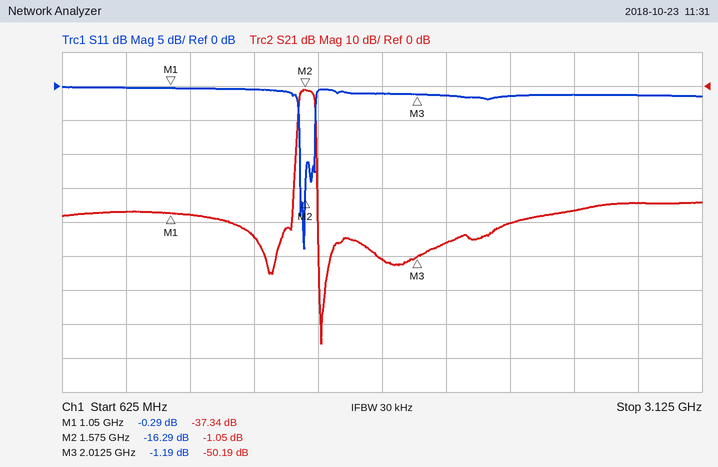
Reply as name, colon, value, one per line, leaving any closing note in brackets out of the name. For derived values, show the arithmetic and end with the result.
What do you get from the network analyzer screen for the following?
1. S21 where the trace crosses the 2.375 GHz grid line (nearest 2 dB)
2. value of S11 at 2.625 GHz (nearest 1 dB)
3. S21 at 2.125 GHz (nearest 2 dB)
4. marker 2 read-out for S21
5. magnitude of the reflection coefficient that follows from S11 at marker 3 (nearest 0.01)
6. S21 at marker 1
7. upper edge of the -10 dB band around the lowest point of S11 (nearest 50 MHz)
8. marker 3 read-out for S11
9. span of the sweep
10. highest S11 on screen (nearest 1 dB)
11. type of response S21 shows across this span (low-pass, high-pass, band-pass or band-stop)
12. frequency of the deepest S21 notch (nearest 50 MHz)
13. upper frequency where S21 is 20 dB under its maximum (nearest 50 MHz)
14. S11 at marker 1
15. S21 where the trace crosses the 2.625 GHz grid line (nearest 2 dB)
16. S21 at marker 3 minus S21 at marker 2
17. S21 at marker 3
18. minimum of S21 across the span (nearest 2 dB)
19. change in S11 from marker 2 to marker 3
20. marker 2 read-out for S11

S21 where the trace crosses the 2.375 GHz grid line: -40 dB
value of S11 at 2.625 GHz: -1 dB
S21 at 2.125 GHz: -46 dB
marker 2 read-out for S21: -1.05 dB
magnitude of the reflection coefficient that follows from S11 at marker 3: 10^(-1.19/20) ≈ 0.87
S21 at marker 1: -37.34 dB
upper edge of the -10 dB band around the lowest point of S11: 1.60 GHz
marker 3 read-out for S11: -1.19 dB
span of the sweep: 2.5 GHz
highest S11 on screen: 0 dB
type of response S21 shows across this span: band-pass
frequency of the deepest S21 notch: 1.65 GHz
upper frequency where S21 is 20 dB under its maximum: 1.60 GHz
S11 at marker 1: -0.29 dB
S21 where the trace crosses the 2.625 GHz grid line: -36 dB
S21 at marker 3 minus S21 at marker 2: -50.19 − (-1.05) = -49.14 dB
S21 at marker 3: -50.19 dB
minimum of S21 across the span: -76 dB
change in S11 from marker 2 to marker 3: -1.19 − (-16.29) = 15.10 dB
marker 2 read-out for S11: -16.29 dB
